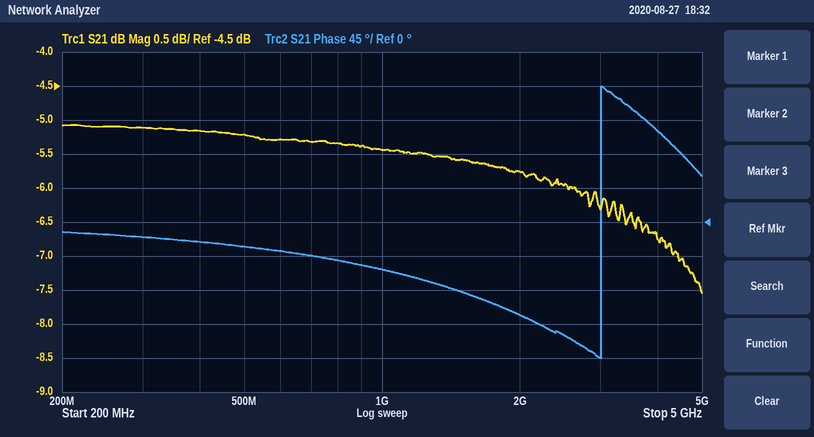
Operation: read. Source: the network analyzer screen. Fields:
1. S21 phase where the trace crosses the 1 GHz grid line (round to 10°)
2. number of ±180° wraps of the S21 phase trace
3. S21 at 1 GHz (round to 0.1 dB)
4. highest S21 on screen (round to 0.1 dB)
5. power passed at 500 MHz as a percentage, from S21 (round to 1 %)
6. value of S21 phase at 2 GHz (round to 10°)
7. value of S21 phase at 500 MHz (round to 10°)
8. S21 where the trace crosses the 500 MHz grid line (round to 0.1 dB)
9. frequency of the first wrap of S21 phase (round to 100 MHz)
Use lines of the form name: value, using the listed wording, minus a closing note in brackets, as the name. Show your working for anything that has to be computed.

S21 phase where the trace crosses the 1 GHz grid line: -60°
number of ±180° wraps of the S21 phase trace: 1
S21 at 1 GHz: -5.4 dB
highest S21 on screen: -5.1 dB
power passed at 500 MHz as a percentage, from S21: 10^(-5.2/10) ≈ 30 %
value of S21 phase at 2 GHz: -120°
value of S21 phase at 500 MHz: -30°
S21 where the trace crosses the 500 MHz grid line: -5.2 dB
frequency of the first wrap of S21 phase: 3.0 GHz
